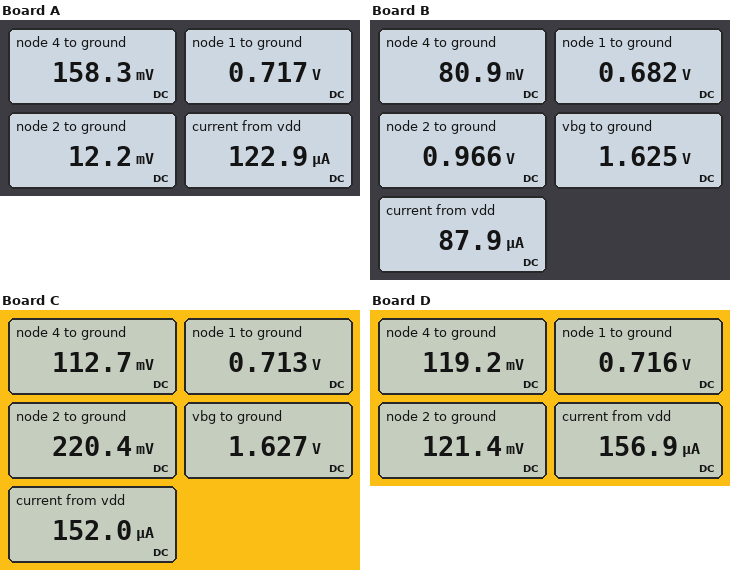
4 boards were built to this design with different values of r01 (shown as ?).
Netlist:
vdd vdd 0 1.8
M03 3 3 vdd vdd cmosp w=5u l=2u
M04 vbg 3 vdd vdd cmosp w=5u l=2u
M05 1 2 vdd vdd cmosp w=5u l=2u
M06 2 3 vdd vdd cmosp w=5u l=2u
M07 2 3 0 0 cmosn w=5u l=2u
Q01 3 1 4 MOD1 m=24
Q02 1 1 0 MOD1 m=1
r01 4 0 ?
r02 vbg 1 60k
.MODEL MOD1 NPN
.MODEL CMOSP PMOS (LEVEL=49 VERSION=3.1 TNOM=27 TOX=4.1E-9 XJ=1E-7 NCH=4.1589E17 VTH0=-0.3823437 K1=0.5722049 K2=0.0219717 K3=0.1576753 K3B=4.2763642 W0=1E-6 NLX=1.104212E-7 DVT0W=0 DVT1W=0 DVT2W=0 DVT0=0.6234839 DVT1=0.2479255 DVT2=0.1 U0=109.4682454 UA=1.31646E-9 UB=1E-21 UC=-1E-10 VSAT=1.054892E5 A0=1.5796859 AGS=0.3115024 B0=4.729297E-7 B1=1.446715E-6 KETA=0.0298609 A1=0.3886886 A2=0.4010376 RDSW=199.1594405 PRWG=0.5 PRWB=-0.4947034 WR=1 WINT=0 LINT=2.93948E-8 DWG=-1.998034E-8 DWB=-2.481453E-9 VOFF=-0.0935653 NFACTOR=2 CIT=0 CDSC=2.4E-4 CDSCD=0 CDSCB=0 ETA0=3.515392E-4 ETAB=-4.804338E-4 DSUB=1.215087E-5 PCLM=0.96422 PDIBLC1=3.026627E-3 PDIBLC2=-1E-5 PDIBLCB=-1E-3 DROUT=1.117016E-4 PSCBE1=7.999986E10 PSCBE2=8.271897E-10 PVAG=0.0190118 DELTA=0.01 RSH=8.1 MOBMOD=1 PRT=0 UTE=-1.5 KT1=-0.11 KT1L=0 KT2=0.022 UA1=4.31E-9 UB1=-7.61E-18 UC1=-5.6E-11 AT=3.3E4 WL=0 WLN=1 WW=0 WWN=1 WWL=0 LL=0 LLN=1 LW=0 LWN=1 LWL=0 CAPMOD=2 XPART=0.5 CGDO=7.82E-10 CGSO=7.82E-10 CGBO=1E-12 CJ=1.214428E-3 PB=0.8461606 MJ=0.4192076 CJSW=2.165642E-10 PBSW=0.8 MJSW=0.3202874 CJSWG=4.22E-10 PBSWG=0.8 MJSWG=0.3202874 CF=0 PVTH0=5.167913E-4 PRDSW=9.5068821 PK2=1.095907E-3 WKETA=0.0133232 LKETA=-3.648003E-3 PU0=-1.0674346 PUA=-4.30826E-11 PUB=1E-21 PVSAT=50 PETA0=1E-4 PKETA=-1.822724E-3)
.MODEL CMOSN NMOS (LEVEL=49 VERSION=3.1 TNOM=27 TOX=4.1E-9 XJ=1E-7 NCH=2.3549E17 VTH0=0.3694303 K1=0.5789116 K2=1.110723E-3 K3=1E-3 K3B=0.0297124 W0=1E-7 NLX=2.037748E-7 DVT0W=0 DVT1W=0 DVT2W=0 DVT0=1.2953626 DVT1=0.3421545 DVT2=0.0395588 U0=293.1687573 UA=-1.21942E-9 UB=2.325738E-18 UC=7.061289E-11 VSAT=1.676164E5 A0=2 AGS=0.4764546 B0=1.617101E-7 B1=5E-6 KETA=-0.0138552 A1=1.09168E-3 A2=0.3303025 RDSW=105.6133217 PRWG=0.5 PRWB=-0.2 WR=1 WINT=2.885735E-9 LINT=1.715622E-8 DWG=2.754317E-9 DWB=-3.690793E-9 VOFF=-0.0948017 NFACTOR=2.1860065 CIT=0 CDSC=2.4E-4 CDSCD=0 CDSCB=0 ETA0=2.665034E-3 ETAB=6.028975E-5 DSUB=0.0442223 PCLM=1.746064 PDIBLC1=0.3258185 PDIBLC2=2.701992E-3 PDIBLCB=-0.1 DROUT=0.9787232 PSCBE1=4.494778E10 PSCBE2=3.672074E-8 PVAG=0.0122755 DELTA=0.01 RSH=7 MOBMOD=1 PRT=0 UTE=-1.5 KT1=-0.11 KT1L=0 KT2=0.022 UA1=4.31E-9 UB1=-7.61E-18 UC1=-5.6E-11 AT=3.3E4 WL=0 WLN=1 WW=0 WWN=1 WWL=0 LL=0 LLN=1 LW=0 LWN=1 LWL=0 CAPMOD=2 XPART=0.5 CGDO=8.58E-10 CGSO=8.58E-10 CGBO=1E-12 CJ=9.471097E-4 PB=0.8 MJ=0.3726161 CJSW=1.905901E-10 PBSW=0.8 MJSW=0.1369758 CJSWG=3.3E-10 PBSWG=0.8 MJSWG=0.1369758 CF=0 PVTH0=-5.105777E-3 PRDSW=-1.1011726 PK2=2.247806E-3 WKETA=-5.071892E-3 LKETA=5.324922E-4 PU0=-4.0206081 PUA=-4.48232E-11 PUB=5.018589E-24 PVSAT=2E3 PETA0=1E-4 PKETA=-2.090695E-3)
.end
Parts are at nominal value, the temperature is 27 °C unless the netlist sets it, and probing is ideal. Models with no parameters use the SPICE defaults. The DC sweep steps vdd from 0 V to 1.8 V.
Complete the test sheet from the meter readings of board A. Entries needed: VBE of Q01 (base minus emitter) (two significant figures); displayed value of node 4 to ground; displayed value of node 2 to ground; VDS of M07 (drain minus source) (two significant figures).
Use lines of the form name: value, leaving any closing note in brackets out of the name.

VBE of Q01 (base minus emitter): 560 mV
displayed value of node 4 to ground: 158.3 mV
displayed value of node 2 to ground: 12.2 mV
VDS of M07 (drain minus source): 12 mV
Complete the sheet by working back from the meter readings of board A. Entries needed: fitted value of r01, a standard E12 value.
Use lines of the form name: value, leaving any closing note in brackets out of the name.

fitted value of r01, a standard E12 value: 27 kΩ
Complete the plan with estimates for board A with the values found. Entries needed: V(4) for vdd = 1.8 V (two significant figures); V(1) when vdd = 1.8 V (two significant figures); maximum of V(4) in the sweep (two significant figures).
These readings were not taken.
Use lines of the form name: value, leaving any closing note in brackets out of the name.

V(4) for vdd = 1.8 V: 160 mV
V(1) when vdd = 1.8 V: 720 mV
maximum of V(4) in the sweep: 160 mV
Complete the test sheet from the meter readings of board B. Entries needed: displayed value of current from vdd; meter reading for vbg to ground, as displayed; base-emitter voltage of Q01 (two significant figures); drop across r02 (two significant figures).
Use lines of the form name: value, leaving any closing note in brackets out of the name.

displayed value of current from vdd: 87.9 µA
meter reading for vbg to ground, as displayed: 1.625 V
base-emitter voltage of Q01: 600 mV
drop across r02: 940 mV
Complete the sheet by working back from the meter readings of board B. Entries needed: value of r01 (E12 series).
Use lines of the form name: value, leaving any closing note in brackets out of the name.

value of r01: 2.7 kΩ
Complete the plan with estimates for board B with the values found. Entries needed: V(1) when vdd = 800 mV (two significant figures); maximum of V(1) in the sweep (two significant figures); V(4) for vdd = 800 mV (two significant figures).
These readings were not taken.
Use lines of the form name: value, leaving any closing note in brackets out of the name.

V(1) when vdd = 800 mV: 600 mV
maximum of V(1) in the sweep: 680 mV
V(4) for vdd = 800 mV: 24 mV
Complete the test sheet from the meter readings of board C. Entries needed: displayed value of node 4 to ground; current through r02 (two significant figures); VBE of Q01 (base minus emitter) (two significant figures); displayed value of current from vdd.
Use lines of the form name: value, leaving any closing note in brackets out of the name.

displayed value of node 4 to ground: 112.7 mV
current through r02: 15 µA
VBE of Q01 (base minus emitter): 600 mV
displayed value of current from vdd: 152.0 µA
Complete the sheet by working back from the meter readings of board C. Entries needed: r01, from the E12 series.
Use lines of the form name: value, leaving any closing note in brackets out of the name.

r01, from the E12 series: 3.9 kΩ
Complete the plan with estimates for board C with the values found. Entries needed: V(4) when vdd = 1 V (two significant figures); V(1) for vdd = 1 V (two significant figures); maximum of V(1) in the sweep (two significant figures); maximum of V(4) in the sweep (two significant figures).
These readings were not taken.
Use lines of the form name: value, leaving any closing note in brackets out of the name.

V(4) when vdd = 1 V: 53 mV
V(1) for vdd = 1 V: 630 mV
maximum of V(1) in the sweep: 710 mV
maximum of V(4) in the sweep: 110 mV
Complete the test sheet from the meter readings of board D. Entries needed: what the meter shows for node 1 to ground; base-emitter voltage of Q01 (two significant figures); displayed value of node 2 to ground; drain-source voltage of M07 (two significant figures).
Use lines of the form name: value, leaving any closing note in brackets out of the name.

what the meter shows for node 1 to ground: 0.716 V
base-emitter voltage of Q01: 600 mV
displayed value of node 2 to ground: 121.4 mV
drain-source voltage of M07: 120 mV
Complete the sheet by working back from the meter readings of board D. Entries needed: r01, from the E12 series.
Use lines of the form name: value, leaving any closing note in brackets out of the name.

r01, from the E12 series: 4.7 kΩ
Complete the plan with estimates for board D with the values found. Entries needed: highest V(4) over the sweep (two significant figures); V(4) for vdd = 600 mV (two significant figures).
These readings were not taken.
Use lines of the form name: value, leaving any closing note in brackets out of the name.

highest V(4) over the sweep: 120 mV
V(4) for vdd = 600 mV: 9.3 mV
